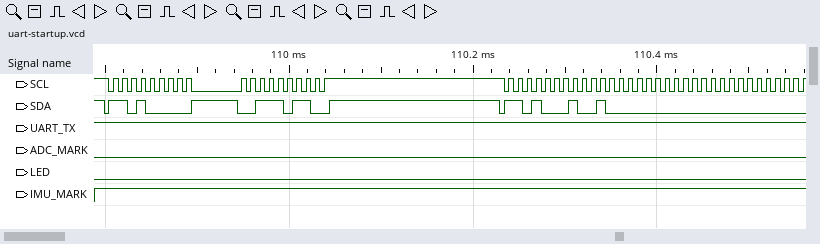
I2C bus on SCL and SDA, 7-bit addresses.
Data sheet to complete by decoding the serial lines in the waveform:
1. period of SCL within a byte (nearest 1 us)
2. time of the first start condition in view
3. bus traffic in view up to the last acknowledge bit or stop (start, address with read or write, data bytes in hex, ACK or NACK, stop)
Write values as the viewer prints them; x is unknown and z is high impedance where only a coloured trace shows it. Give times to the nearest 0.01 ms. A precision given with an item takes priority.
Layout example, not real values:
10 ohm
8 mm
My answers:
10 us
109.8 ms
start, address 68 write ACK, 3B ACK, stop, start, address 68 read ACK, 40 ACK, 00 ACK
